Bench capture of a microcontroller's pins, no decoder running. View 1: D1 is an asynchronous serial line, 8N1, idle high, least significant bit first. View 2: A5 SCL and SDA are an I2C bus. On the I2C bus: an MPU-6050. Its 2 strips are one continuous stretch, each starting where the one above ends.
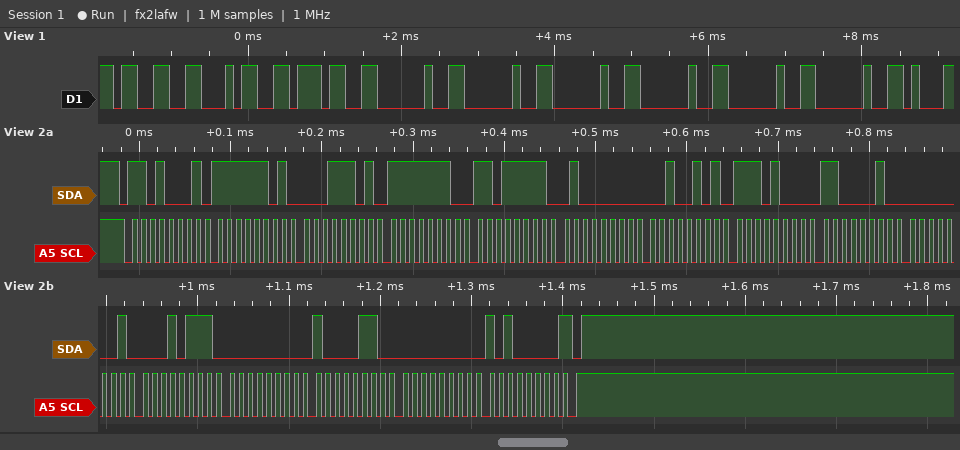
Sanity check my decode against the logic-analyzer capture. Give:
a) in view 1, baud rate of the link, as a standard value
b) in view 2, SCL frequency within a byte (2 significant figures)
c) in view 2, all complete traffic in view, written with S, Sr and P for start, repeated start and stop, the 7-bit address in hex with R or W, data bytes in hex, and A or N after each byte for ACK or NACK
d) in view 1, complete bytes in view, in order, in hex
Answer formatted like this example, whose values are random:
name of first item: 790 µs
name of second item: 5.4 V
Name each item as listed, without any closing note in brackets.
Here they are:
in view 1, baud rate of the link, as a standard value: 9600 baud
in view 2, SCL frequency within a byte: 100 kHz
in view 2, all complete traffic in view, written with S, Sr and P for start, repeated start and stop, the 7-bit address in hex with R or W, data bytes in hex, and A or N after each byte for ACK or NACK: S 68R A FD A 1D A FE A DF A 40 A 25 A E8 A C2 A 01 A 17 A 00 A 86 A 00 A A0 N P
in view 1, complete bytes in view, in order, in hex: 33 34 37 20 20 20 20 20 20
